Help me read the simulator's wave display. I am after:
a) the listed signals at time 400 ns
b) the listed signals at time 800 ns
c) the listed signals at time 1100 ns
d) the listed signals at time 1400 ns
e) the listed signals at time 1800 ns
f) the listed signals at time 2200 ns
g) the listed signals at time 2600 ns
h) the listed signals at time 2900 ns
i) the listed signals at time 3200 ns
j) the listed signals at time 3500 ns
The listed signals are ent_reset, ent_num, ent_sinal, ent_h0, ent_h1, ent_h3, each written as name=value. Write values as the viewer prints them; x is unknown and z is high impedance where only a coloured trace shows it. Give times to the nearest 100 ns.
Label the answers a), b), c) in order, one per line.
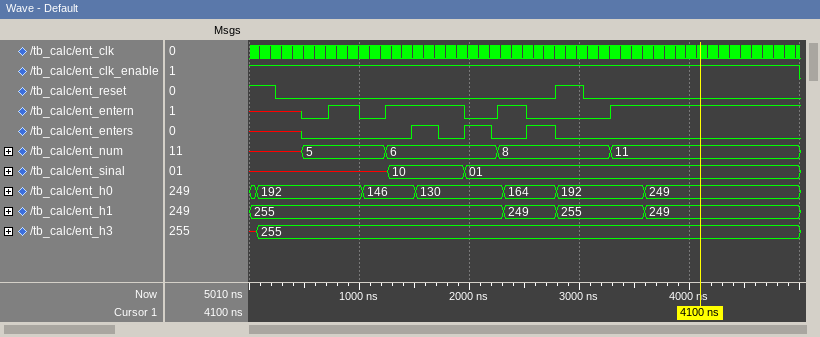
a) ent_reset=0, ent_num=x, ent_sinal=x, ent_h0=192, ent_h1=255, ent_h3=255
b) ent_reset=0, ent_num=5, ent_sinal=x, ent_h0=192, ent_h1=255, ent_h3=255
c) ent_reset=0, ent_num=5, ent_sinal=x, ent_h0=146, ent_h1=255, ent_h3=255
d) ent_reset=0, ent_num=6, ent_sinal=10, ent_h0=146, ent_h1=255, ent_h3=255
e) ent_reset=0, ent_num=6, ent_sinal=10, ent_h0=130, ent_h1=255, ent_h3=255
f) ent_reset=0, ent_num=6, ent_sinal=01, ent_h0=130, ent_h1=255, ent_h3=255
g) ent_reset=0, ent_num=8, ent_sinal=01, ent_h0=164, ent_h1=249, ent_h3=255
h) ent_reset=1, ent_num=8, ent_sinal=01, ent_h0=192, ent_h1=255, ent_h3=255
i) ent_reset=0, ent_num=8, ent_sinal=01, ent_h0=192, ent_h1=255, ent_h3=255
j) ent_reset=0, ent_num=11, ent_sinal=01, ent_h0=192, ent_h1=255, ent_h3=255
